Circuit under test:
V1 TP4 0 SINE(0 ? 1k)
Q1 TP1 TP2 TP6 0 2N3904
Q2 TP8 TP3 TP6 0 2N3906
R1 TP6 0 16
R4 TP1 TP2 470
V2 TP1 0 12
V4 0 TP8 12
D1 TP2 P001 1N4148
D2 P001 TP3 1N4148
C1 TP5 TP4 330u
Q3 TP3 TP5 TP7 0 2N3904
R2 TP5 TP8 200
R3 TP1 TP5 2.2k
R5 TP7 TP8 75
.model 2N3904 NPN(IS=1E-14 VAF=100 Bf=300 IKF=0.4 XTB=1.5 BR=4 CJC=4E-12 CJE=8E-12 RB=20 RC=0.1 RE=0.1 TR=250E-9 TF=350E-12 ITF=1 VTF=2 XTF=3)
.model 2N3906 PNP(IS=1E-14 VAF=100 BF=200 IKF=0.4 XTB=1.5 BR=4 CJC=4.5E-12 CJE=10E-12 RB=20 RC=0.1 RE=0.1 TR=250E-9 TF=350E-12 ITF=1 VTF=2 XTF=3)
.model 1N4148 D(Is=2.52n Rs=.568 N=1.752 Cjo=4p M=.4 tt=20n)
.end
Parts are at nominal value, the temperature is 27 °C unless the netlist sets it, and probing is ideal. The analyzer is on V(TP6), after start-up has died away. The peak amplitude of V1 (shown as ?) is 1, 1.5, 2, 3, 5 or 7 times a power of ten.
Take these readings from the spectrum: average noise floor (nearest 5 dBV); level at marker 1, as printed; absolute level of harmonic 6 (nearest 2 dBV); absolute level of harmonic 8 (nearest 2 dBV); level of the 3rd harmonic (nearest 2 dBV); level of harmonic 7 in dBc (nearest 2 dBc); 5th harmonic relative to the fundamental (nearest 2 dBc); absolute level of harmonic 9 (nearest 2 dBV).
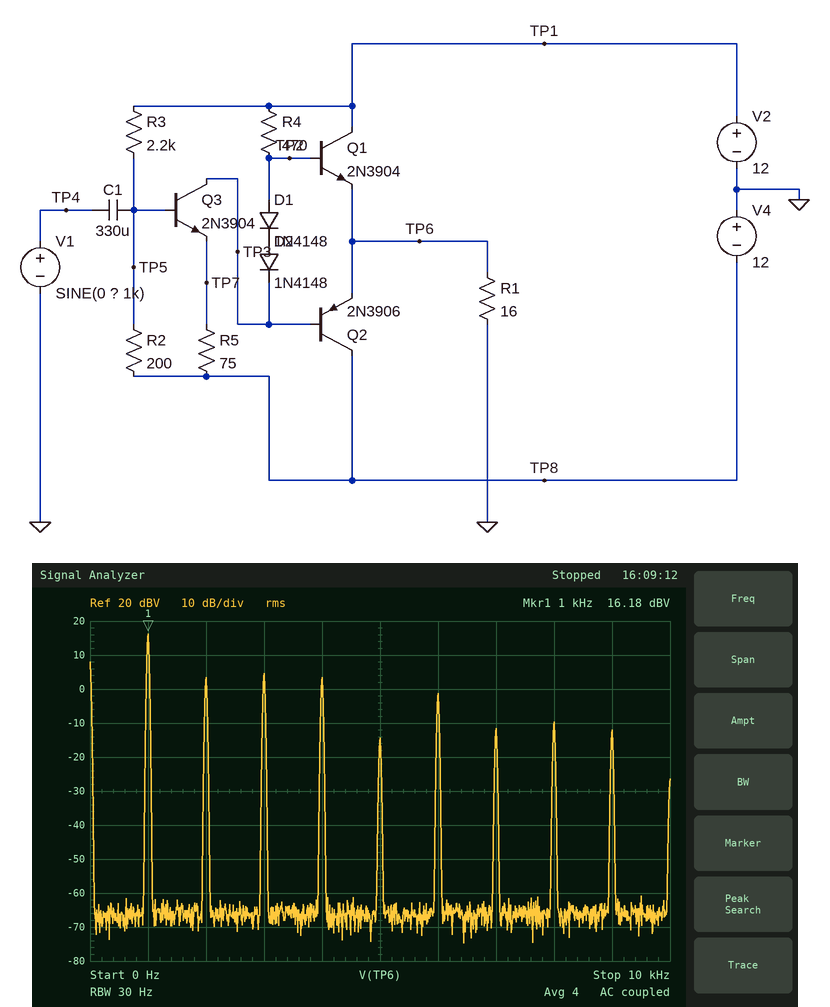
-65 dBV
16.18 dBV
-2 dBV
-10 dBV
4 dBV
-28 dBc
-30 dBc
-12 dBV
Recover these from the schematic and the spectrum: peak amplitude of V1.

7 V
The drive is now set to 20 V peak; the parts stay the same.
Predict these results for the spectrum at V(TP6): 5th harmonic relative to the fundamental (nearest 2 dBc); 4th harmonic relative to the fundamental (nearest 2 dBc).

-36 dBc
-8 dBc
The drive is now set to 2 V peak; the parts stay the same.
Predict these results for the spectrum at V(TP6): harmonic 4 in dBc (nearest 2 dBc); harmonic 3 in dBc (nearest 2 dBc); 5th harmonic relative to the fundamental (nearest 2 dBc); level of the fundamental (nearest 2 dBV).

-34 dBc
-22 dBc
-58 dBc
16 dBV
